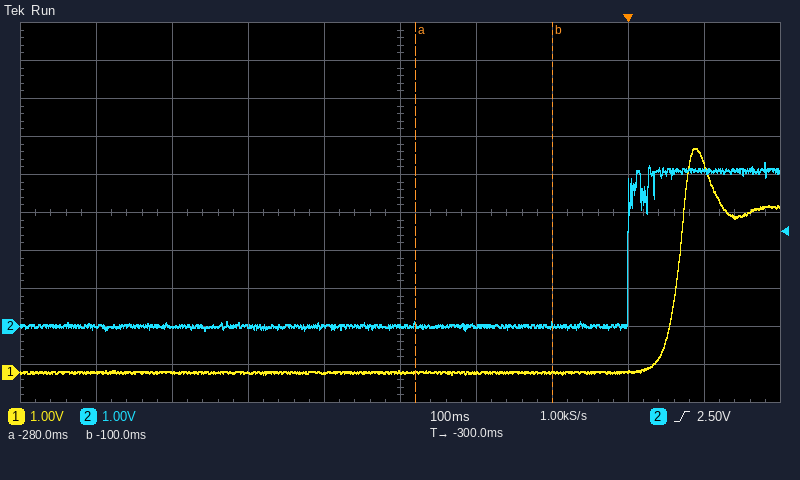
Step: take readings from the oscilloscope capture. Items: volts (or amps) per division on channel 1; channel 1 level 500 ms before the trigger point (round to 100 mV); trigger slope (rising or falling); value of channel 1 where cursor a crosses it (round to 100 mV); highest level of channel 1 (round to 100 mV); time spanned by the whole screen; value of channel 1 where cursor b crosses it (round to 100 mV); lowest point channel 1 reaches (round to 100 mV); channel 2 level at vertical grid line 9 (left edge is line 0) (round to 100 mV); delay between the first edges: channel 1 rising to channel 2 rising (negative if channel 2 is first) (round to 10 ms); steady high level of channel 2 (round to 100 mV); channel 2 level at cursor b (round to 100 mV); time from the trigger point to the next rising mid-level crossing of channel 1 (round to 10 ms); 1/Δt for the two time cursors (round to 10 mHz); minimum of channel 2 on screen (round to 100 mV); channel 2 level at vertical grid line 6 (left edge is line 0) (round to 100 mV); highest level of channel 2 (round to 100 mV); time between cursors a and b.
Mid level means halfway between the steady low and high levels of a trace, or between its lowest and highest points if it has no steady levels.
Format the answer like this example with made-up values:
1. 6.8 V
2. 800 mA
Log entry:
1. 1 V
2. 0.0 V
3. rising
4. 0.0 V
5. 5.9 V
6. 1 s
7. 0.0 V
8. -100 mV
9. 4.1 V
10. -70 ms
11. 4.1 V
12. 0.0 V
13. 70 ms
14. 5.56 Hz
15. -100 mV
16. 0.0 V
17. 4.3 V
18. 180 ms
